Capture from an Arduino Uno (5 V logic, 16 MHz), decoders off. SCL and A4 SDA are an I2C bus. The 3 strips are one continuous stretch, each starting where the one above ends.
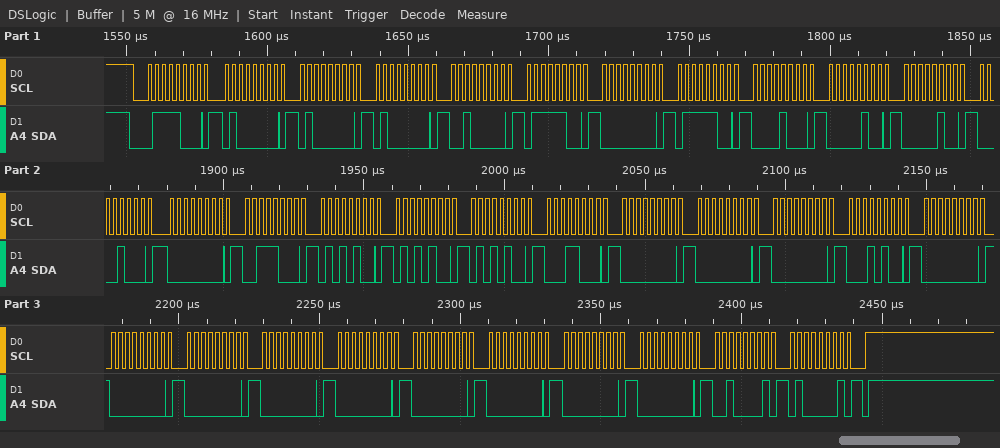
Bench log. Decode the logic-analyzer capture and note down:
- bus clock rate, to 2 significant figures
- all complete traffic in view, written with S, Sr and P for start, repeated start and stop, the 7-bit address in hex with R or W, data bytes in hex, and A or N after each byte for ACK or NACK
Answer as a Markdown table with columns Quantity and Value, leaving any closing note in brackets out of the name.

| Quantity | Value |
|---|---|
| bus clock rate, to 2 significant figures | 400 kHz |
| all complete traffic in view, written with S, Sr and P for start, repeated start and stop, the 7-bit address in hex with R or W, data bytes in hex, and A or N after each byte for ACK or NACK | S 3CW A 40 A 40 A 40 A 20 A 7C A 00 A 7C A 08 A 04 A 04 A 08 A 00 A 38 A 54 A 54 A 54 A 18 A 00 A 00 A 00 A 14 A 00 A 00 A 00 A 00 A 00 A 00 A 00 A 00 A 00 A 21 A 41 A P |
